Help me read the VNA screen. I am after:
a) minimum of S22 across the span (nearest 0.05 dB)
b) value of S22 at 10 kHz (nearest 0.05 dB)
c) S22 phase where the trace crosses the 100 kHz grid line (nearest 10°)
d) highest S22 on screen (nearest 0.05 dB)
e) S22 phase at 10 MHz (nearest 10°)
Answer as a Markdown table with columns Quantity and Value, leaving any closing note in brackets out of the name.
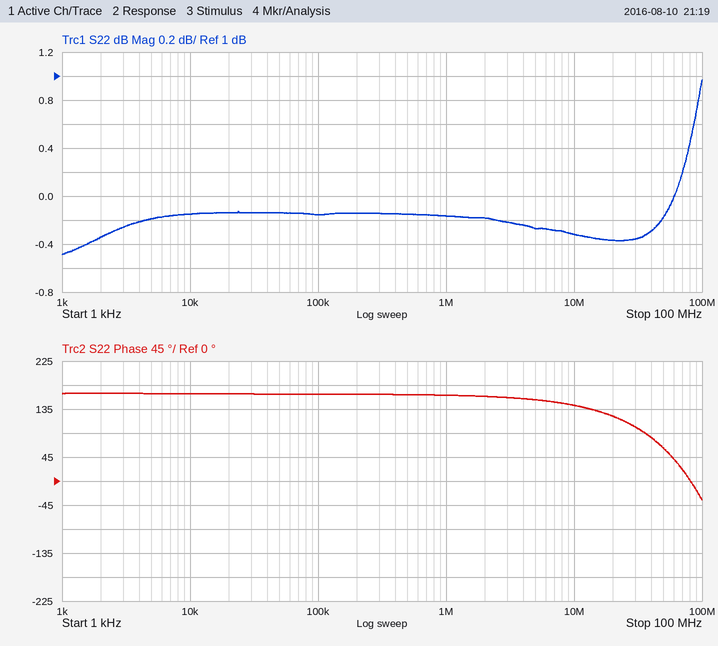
| Quantity | Value |
|---|---|
| minimum of S22 across the span | -0.50 dB |
| value of S22 at 10 kHz | -0.15 dB |
| S22 phase where the trace crosses the 100 kHz grid line | 160° |
| highest S22 on screen | 0.95 dB |
| S22 phase at 10 MHz | 140° |
